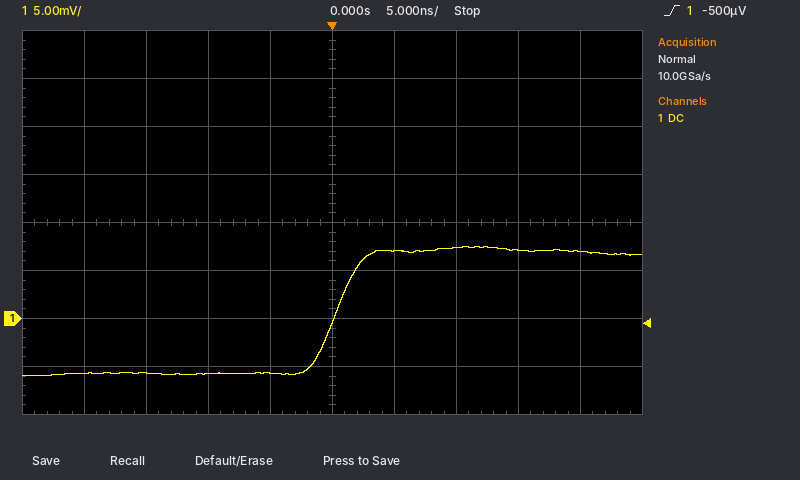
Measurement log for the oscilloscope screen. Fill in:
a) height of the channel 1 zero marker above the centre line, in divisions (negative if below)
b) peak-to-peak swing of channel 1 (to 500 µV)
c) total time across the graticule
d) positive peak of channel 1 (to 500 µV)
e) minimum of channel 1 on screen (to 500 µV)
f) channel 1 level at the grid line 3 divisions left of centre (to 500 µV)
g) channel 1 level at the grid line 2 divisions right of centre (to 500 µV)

-2.0 div
13.5 mV
50 ns
7.5 mV
-6.0 mV
-5.5 mV
7.5 mV
